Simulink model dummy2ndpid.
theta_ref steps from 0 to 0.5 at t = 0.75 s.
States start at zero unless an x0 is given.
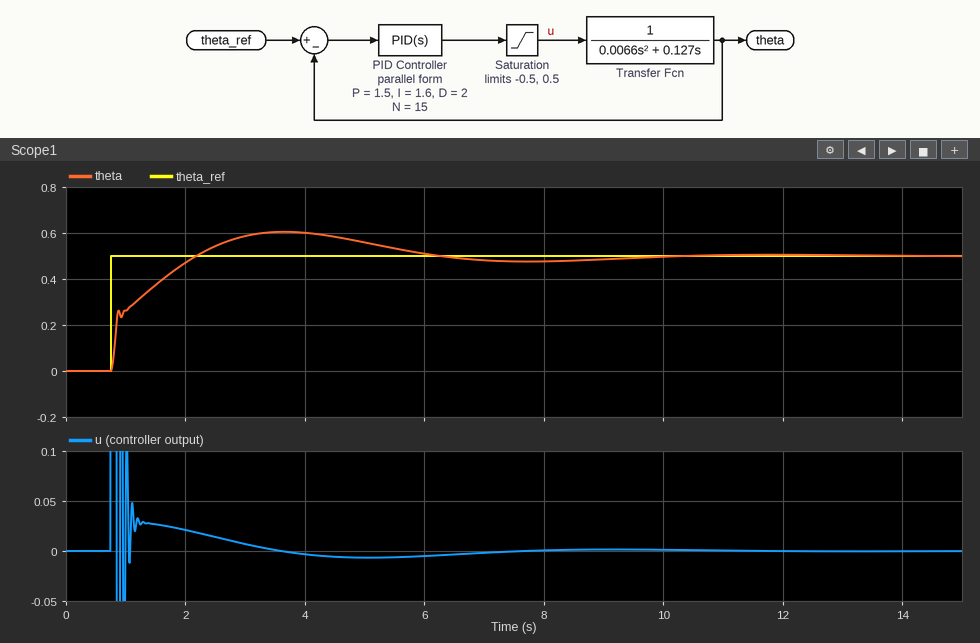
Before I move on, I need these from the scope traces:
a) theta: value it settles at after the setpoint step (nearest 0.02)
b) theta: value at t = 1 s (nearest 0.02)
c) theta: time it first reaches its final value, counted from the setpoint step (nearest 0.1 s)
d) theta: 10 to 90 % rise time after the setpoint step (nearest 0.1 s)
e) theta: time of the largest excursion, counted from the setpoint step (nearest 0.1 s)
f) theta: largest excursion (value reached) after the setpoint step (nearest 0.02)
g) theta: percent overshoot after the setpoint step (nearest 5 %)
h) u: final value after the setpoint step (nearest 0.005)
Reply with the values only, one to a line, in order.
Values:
0.50
0.26
1.4 s
1.1 s
2.9 s
0.60
20 %
0.000
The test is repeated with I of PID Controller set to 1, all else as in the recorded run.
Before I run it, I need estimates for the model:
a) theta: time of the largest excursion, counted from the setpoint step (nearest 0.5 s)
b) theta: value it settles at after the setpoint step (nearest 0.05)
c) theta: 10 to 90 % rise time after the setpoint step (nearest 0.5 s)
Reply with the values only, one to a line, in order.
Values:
3.5 s
0.50
1.5 s
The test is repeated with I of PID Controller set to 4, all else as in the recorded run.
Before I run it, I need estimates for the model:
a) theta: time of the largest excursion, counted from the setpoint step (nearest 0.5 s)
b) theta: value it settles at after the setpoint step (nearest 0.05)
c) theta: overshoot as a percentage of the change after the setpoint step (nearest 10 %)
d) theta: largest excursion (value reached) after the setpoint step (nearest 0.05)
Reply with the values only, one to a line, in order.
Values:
2.0 s
0.50
30 %
0.65
